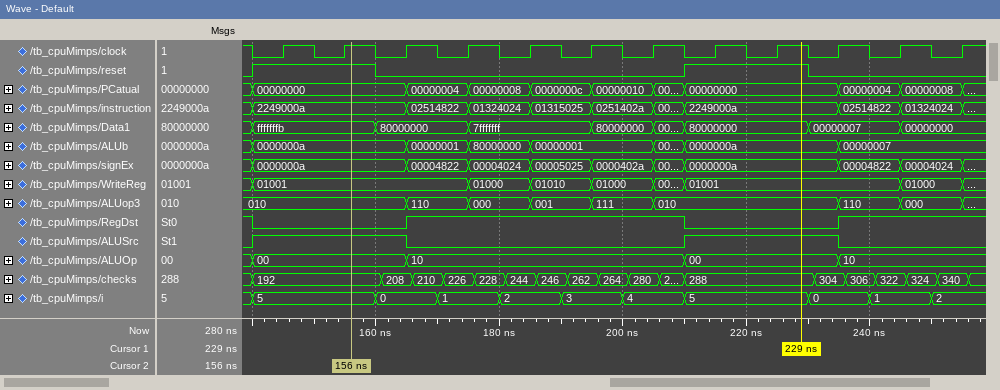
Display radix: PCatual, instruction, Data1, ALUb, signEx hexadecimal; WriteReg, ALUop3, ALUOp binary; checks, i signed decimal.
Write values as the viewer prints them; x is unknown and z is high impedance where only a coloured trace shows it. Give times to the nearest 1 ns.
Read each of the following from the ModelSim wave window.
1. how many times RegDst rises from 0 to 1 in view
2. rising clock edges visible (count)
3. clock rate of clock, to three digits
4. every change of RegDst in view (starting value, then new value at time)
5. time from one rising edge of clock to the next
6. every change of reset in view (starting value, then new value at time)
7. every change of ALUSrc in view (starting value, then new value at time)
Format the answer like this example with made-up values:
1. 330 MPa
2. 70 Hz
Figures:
1. 2
2. 12
3. 100 MHz
4. 1, 0 at 140 ns, 1 at 165 ns, 0 at 210 ns, 1 at 235 ns
5. 10 ns
6. 0, 1 at 140 ns, 0 at 160 ns, 1 at 210 ns, 0 at 230 ns
7. 0, 1 at 140 ns, 0 at 165 ns, 1 at 210 ns, 0 at 235 ns
